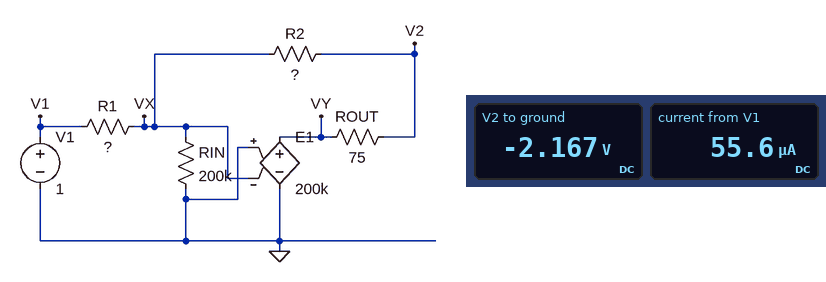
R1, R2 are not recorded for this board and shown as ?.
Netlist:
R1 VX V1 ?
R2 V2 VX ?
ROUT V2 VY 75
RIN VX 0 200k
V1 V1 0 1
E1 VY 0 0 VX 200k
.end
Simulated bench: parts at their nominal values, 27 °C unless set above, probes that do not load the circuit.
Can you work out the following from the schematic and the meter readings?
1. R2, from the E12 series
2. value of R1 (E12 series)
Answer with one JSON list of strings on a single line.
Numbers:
["39 kΩ", "18 kΩ"]
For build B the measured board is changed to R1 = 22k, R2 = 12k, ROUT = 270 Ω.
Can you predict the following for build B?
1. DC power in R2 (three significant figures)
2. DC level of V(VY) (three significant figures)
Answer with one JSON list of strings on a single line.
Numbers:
["24.8 µW", "-558 mV"]
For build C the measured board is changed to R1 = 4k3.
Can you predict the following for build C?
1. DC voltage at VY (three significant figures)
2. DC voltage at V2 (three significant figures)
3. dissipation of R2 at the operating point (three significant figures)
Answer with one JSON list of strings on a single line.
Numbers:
["-9.09 V", "-9.07 V", "2.11 mW"]
